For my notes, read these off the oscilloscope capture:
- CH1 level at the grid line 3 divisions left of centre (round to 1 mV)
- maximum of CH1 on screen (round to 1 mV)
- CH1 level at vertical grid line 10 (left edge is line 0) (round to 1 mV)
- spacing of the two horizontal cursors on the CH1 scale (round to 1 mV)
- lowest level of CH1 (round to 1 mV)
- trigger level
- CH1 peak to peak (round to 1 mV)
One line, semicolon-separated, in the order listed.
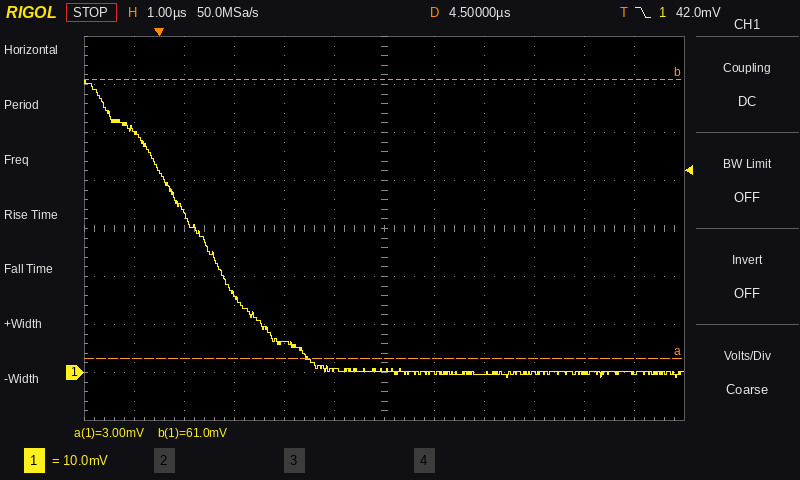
16 mV; 61 mV; 0 mV; 58 mV; -1 mV; 42.0 mV; 62 mV
